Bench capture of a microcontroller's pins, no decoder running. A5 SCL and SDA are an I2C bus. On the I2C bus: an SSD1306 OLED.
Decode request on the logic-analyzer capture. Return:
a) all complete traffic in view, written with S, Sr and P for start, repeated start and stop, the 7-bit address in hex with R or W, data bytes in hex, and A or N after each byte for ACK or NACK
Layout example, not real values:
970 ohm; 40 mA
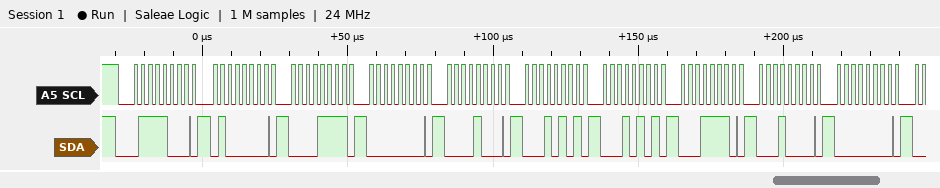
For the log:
S 3CW A 40 A 0F A 00 A 08 A 15 A 15 A 1E A 10 A 00 A
